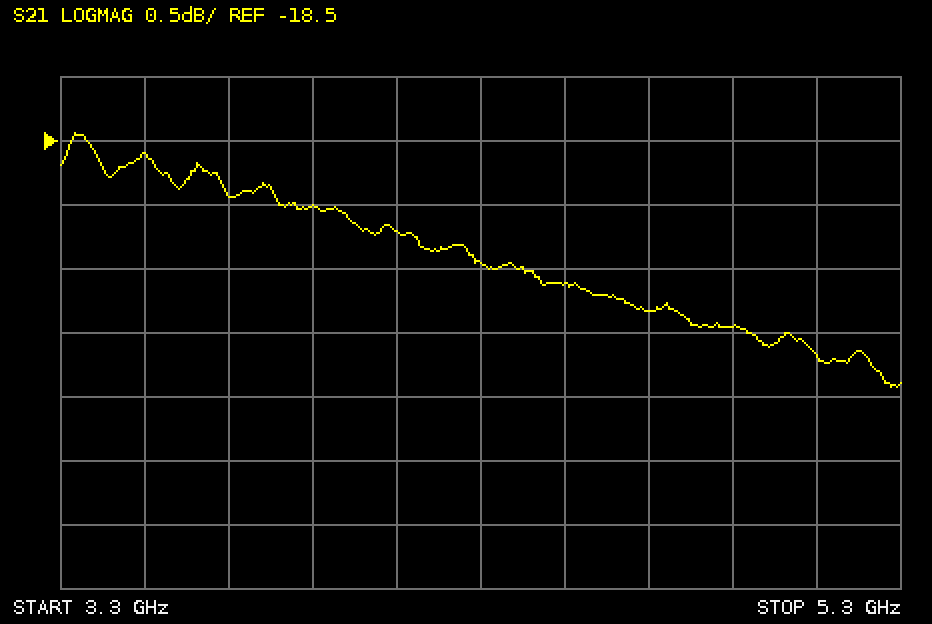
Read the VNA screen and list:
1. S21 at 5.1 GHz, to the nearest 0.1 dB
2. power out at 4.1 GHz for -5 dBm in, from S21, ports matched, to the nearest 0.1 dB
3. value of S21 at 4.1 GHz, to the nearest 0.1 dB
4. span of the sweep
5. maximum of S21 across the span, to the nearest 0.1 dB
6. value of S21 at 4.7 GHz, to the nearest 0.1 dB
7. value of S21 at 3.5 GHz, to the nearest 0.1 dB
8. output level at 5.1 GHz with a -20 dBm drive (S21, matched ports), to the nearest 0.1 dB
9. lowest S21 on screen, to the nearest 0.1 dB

-20.2 dB
-24.2 dBm
-19.2 dB
2 GHz
-18.4 dB
-19.8 dB
-18.6 dB
-40.2 dBm
-20.4 dB
